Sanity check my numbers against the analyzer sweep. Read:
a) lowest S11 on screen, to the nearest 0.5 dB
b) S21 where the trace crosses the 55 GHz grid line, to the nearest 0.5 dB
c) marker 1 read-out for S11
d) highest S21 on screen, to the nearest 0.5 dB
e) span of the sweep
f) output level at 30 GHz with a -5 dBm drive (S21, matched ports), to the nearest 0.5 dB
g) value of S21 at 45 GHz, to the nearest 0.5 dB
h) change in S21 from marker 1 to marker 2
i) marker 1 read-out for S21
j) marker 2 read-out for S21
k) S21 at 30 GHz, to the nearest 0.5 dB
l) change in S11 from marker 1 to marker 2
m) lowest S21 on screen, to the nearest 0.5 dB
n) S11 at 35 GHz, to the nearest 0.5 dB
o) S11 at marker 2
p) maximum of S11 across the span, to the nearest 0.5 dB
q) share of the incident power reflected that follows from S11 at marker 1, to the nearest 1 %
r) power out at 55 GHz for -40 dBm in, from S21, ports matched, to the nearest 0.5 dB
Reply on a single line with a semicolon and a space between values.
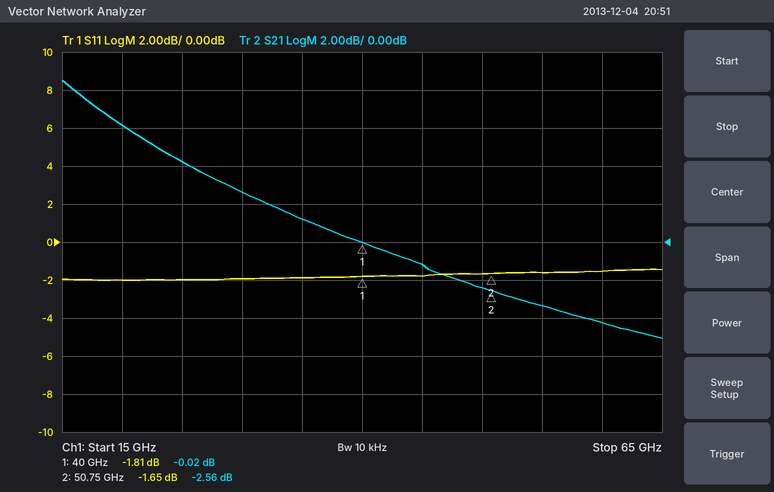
-2.0 dB; -3.5 dB; -1.81 dB; 8.5 dB; 50 GHz; -2.5 dBm; -1.0 dB; -2.54 dB; -0.02 dB; -2.56 dB; 2.5 dB; 0.16 dB; -5.0 dB; -2.0 dB; -1.65 dB; -1.5 dB; 66 %; -43.5 dBm
